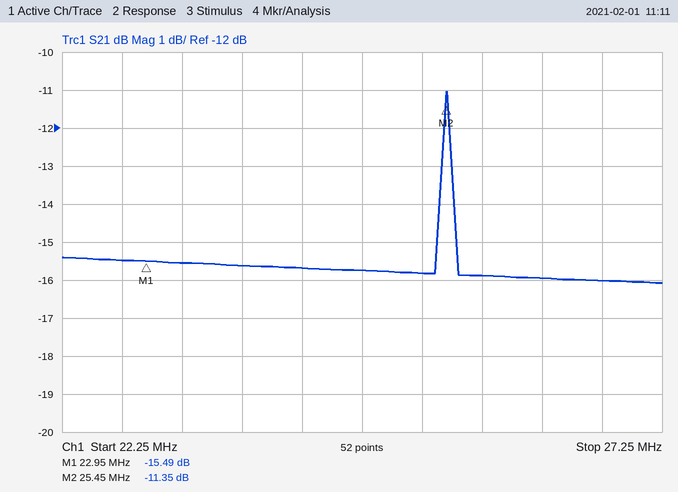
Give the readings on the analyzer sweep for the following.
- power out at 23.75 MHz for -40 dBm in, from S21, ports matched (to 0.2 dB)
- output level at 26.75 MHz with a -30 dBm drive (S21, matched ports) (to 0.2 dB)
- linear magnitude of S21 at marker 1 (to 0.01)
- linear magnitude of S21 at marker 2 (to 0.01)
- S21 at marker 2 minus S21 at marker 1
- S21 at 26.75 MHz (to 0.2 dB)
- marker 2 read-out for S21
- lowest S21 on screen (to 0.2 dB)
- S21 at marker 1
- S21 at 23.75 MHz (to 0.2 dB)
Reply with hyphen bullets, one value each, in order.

- -55.6 dBm
- -46.0 dBm
- 0.17
- 0.27
- 4.14 dB
- -16.0 dB
- -11.35 dB
- -16.0 dB
- -15.49 dB
- -15.6 dB
